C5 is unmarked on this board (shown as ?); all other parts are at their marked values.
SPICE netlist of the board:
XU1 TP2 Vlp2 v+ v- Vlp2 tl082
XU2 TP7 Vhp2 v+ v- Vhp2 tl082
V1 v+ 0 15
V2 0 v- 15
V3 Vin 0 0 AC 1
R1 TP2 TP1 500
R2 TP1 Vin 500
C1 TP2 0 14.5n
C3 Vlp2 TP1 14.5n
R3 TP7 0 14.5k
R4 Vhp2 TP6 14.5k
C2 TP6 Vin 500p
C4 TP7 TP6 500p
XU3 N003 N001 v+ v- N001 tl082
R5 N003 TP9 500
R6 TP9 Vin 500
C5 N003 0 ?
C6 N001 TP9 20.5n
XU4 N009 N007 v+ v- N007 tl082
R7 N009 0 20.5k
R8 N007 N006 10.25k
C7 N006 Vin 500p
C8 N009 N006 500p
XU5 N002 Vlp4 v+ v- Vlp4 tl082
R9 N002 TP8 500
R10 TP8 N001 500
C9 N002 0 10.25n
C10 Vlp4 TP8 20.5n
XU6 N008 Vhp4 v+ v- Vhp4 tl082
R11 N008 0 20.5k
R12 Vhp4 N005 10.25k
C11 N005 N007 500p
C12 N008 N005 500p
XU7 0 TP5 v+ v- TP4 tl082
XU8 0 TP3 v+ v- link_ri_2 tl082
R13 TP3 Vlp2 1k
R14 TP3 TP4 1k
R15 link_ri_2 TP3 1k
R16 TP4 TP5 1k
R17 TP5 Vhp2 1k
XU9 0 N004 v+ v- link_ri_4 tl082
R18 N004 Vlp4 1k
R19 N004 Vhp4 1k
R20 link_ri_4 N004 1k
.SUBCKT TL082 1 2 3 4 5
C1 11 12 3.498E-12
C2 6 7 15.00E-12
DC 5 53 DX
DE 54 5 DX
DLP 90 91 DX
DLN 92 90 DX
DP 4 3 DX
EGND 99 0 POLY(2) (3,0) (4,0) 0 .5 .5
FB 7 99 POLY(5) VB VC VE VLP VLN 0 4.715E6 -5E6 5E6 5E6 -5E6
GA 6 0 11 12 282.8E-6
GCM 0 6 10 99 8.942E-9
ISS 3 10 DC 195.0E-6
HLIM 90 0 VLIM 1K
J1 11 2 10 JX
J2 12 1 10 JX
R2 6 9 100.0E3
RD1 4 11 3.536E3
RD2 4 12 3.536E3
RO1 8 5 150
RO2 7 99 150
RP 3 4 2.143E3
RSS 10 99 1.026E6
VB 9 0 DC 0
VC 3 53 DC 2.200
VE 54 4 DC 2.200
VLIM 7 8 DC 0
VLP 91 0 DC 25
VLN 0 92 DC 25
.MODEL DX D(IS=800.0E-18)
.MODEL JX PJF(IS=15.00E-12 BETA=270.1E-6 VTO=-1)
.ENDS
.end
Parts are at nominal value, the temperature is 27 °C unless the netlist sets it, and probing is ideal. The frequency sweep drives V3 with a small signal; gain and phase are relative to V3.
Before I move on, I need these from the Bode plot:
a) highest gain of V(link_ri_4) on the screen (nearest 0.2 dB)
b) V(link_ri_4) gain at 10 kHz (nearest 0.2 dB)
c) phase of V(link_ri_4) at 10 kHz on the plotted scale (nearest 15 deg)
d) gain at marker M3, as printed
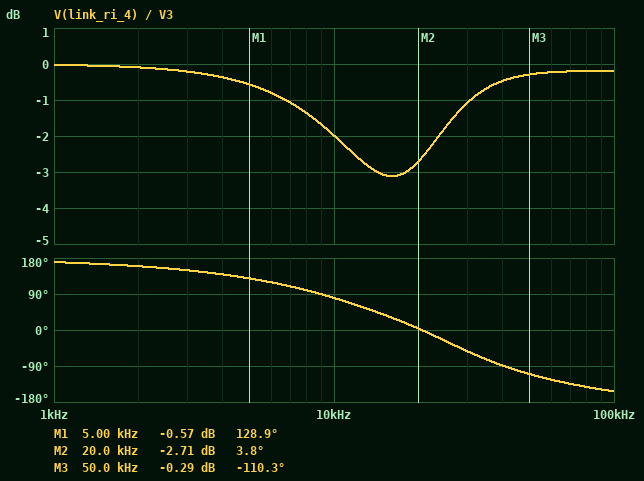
0 dB
-2.0 dB
75 deg
-0.29 dB
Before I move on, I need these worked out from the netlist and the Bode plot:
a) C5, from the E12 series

18 nF
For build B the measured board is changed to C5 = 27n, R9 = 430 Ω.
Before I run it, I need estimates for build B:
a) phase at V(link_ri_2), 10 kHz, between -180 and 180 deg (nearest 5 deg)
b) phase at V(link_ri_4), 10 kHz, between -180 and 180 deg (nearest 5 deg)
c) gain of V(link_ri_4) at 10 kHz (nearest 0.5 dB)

130 deg
70 deg
-4.5 dB
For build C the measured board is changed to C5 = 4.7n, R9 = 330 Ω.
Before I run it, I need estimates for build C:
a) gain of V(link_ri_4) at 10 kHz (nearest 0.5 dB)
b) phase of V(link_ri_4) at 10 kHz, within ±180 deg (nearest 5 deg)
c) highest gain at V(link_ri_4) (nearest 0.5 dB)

0.5 dB
130 deg
2.5 dB
